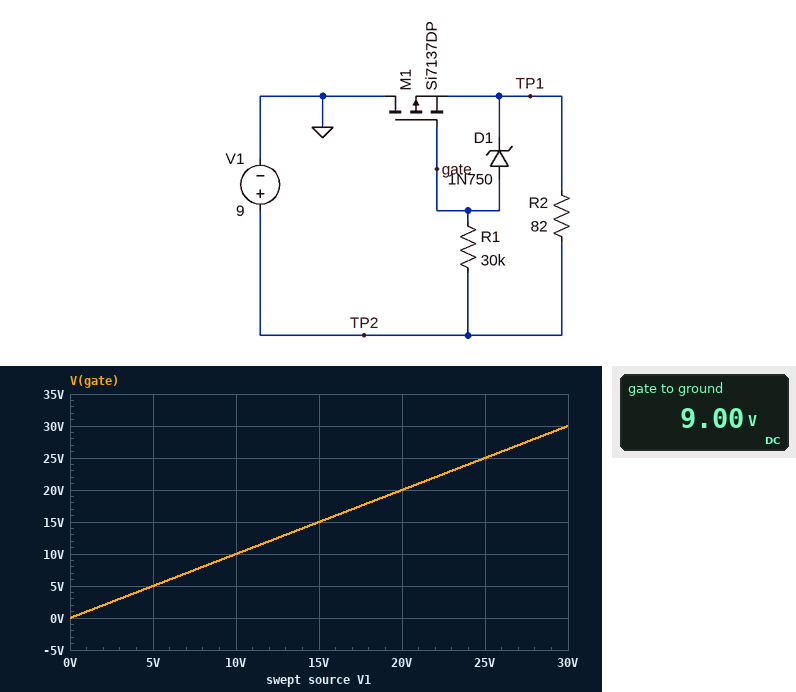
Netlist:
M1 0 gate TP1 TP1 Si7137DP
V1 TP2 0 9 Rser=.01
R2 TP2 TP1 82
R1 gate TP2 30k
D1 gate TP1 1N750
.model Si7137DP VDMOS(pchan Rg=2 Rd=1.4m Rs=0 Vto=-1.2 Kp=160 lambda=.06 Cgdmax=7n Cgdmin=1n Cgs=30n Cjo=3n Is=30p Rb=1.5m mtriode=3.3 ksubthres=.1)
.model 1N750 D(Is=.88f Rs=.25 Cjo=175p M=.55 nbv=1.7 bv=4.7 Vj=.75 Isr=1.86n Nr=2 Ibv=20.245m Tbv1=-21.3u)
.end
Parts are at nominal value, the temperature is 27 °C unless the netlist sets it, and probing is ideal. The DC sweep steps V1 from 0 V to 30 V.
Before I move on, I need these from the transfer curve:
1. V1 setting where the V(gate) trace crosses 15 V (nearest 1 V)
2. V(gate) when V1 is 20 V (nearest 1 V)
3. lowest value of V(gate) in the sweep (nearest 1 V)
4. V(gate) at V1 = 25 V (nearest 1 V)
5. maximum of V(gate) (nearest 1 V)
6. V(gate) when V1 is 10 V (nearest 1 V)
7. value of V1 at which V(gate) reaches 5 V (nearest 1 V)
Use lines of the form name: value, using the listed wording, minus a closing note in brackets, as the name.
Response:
V1 setting where the V(gate) trace crosses 15 V: 15 V
V(gate) when V1 is 20 V: 20 V
lowest value of V(gate) in the sweep: 0 V
V(gate) at V1 = 25 V: 25 V
maximum of V(gate): 30 V
V(gate) when V1 is 10 V: 10 V
value of V1 at which V(gate) reaches 5 V: 5 V
